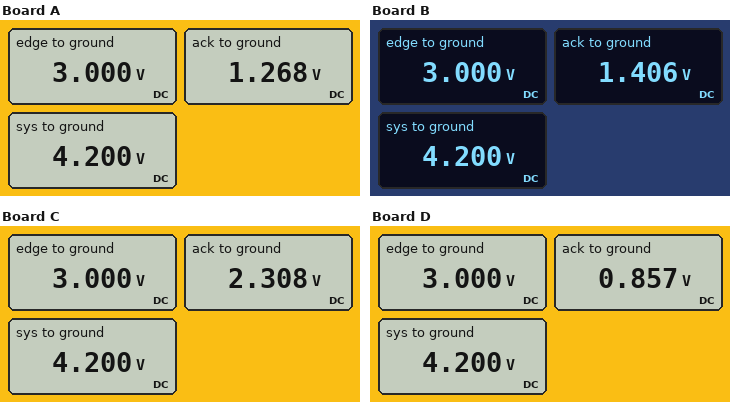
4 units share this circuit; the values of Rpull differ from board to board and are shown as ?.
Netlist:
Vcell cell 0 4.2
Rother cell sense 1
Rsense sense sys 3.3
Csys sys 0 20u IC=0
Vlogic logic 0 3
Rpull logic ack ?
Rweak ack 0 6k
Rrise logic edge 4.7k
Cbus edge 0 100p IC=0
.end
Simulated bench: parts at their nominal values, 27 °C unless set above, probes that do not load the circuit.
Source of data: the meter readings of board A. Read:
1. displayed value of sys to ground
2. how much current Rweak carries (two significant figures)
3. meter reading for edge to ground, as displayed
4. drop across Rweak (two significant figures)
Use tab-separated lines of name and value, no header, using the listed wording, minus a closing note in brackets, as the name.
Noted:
displayed value of sys to ground	4.200 V
how much current Rweak carries	210 µA
meter reading for edge to ground, as displayed	3.000 V
drop across Rweak	1.3 V
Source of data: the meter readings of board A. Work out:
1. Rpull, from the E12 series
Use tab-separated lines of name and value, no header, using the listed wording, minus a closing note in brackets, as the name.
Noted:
Rpull, from the E12 series	8.2 kΩ
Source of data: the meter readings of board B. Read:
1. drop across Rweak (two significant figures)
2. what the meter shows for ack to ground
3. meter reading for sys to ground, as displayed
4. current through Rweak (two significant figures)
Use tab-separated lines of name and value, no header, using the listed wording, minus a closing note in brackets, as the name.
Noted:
drop across Rweak	1.4 V
what the meter shows for ack to ground	1.406 V
meter reading for sys to ground, as displayed	4.200 V
current through Rweak	230 µA
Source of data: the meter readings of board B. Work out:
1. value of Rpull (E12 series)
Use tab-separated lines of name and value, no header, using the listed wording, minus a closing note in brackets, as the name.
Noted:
value of Rpull	6.8 kΩ
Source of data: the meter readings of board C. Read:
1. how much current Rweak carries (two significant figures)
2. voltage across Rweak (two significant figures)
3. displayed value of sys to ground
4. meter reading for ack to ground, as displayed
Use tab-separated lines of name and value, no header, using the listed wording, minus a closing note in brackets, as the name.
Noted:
how much current Rweak carries	380 µA
voltage across Rweak	2.3 V
displayed value of sys to ground	4.200 V
meter reading for ack to ground, as displayed	2.308 V
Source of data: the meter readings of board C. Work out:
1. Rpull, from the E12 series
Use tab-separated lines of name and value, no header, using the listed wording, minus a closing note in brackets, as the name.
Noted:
Rpull, from the E12 series	1.8 kΩ
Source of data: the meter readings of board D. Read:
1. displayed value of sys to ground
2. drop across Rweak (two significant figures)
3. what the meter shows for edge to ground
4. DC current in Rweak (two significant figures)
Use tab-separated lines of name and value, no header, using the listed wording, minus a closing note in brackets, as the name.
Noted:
displayed value of sys to ground	4.200 V
drop across Rweak	860 mV
what the meter shows for edge to ground	3.000 V
DC current in Rweak	140 µA
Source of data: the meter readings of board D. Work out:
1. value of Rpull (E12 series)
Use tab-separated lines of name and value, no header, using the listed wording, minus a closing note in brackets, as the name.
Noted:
value of Rpull	15 kΩ
